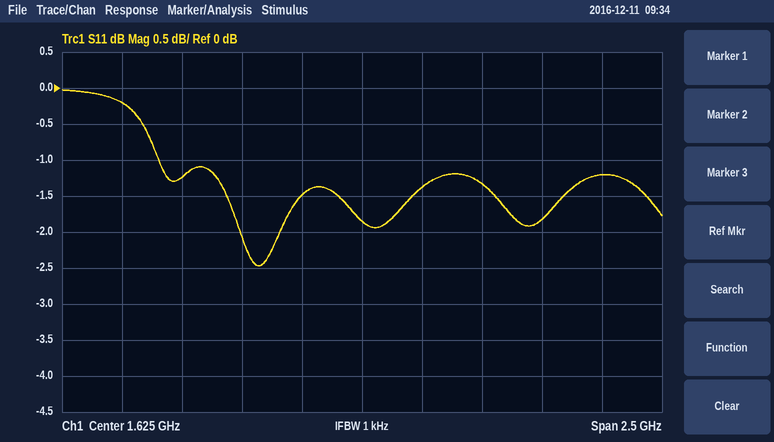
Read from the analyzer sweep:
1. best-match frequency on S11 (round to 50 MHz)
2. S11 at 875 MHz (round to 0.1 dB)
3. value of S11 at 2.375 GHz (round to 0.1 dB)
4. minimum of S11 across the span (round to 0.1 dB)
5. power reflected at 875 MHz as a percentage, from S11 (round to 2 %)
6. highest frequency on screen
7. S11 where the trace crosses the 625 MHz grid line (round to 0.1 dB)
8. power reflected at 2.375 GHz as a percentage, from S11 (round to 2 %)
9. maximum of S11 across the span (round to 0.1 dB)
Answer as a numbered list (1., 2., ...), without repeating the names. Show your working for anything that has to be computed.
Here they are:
1. 1.20 GHz
2. -1.2 dB
3. -1.8 dB
4. -2.5 dB
5. 10^(-1.2/10) ≈ 76 %
6. 2.875 GHz
7. -0.2 dB
8. 10^(-1.8/10) ≈ 66 %
9. 0.0 dB
